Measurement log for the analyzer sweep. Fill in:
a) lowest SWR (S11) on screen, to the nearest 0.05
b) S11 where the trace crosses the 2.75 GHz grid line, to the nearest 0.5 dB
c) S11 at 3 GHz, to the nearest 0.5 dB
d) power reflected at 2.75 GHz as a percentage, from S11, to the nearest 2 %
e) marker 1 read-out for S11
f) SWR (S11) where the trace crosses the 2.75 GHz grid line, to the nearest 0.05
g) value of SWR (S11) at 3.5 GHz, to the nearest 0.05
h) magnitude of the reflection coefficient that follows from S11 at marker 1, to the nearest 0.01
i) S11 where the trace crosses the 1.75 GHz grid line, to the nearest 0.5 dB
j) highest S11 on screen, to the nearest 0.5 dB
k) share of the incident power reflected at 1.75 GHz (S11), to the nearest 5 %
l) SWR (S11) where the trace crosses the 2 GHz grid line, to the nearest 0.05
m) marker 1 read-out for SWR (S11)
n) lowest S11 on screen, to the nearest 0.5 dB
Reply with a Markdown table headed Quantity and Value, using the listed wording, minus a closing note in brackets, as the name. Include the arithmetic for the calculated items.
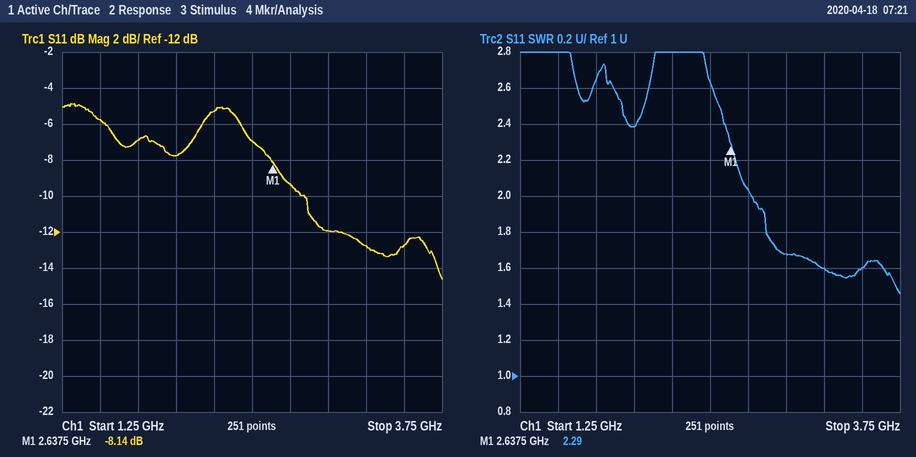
| Quantity | Value |
|---|---|
| lowest SWR (S11) on screen, to the nearest 0.05 | 1.45 |
| S11 where the trace crosses the 2.75 GHz grid line, to the nearest 0.5 dB | -9.5 dB |
| S11 at 3 GHz, to the nearest 0.5 dB | -12.0 dB |
| power reflected at 2.75 GHz as a percentage, from S11, to the nearest 2 % | 10^(-9.5/10) ≈ 11.2 %, so 12 % to the nearest 2 % |
| marker 1 read-out for S11 | -8.14 dB |
| SWR (S11) where the trace crosses the 2.75 GHz grid line, to the nearest 0.05 | 2.05 |
| value of SWR (S11) at 3.5 GHz, to the nearest 0.05 | 1.60 |
| magnitude of the reflection coefficient that follows from S11 at marker 1, to the nearest 0.01 | 10^(-8.14/20) ≈ 0.39 |
| S11 where the trace crosses the 1.75 GHz grid line, to the nearest 0.5 dB | -7.0 dB |
| highest S11 on screen, to the nearest 0.5 dB | -5.0 dB |
| share of the incident power reflected at 1.75 GHz (S11), to the nearest 5 % | 10^(-7/10) ≈ 20 % |
| SWR (S11) where the trace crosses the 2 GHz grid line, to the nearest 0.05 | 2.40 |
| marker 1 read-out for SWR | 2.29 |
| lowest S11 on screen, to the nearest 0.5 dB | -14.5 dB |
